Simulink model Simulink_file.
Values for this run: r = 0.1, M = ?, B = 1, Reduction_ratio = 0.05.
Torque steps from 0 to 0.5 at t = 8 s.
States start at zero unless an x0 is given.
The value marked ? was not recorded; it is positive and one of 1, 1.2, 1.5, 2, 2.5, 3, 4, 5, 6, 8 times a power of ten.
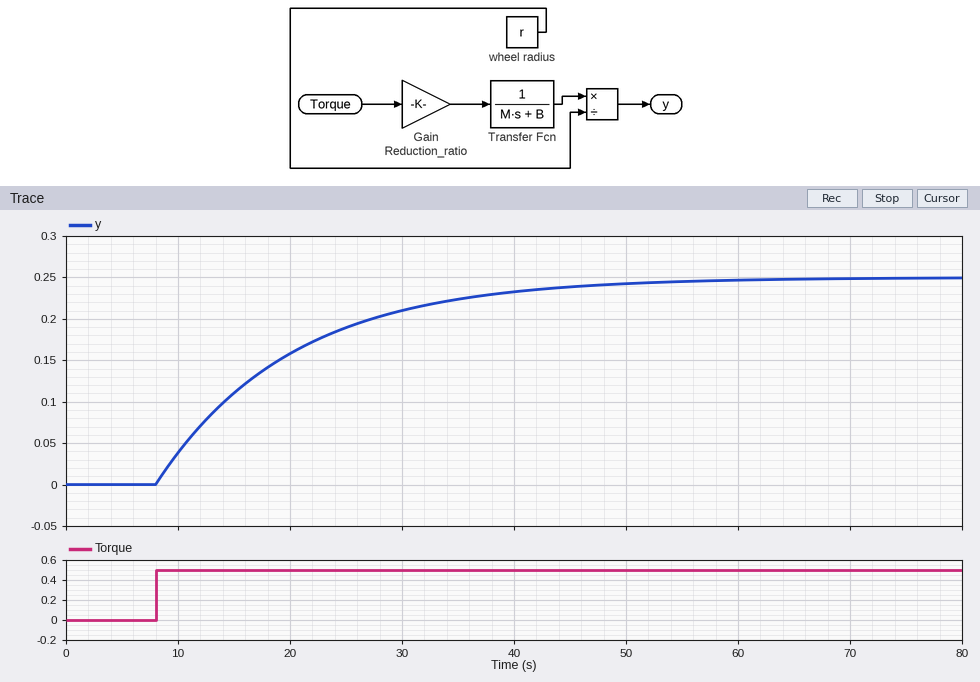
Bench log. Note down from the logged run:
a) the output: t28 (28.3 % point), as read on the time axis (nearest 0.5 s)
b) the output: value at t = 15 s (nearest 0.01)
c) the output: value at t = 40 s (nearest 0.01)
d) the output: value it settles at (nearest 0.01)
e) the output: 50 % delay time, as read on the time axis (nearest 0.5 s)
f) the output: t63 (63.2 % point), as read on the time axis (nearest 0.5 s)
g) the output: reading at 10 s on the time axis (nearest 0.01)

12.0 s
0.11
0.23
0.25
16.5 s
20.0 s
0.04
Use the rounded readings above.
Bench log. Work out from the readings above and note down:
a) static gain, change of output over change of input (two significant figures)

0.50
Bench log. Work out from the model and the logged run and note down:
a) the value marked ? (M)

12
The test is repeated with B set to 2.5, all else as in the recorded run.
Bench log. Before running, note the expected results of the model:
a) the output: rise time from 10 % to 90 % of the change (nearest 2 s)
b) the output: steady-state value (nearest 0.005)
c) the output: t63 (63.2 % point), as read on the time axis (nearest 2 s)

10 s
0.100
12 s
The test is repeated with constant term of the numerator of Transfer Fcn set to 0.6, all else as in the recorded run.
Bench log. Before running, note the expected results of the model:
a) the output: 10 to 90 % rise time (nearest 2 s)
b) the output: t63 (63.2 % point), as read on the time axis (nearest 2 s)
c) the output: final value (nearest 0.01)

26 s
20 s
0.15
